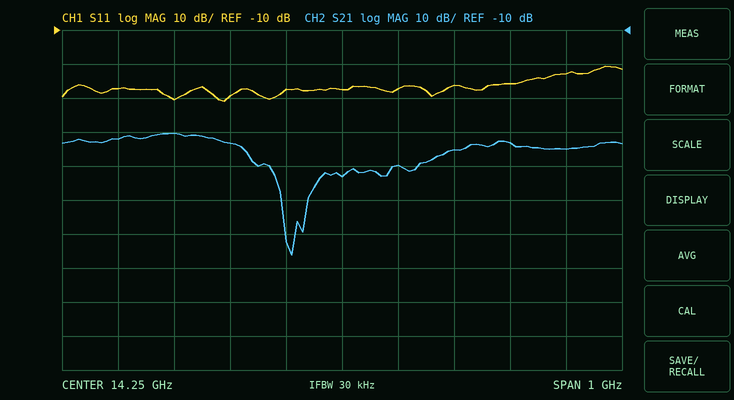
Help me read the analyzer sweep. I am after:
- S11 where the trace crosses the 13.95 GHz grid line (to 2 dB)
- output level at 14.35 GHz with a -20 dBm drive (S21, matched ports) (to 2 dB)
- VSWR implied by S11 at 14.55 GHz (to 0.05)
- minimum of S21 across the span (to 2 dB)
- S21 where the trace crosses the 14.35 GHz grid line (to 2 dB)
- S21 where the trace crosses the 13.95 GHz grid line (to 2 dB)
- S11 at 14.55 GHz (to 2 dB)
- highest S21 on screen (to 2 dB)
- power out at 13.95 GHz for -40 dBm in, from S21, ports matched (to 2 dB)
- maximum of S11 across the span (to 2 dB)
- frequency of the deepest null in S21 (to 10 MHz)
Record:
-30 dB
-70 dBm
1.10
-76 dB
-50 dB
-40 dB
-26 dB
-40 dB
-80 dBm
-20 dB
14.16 GHz
